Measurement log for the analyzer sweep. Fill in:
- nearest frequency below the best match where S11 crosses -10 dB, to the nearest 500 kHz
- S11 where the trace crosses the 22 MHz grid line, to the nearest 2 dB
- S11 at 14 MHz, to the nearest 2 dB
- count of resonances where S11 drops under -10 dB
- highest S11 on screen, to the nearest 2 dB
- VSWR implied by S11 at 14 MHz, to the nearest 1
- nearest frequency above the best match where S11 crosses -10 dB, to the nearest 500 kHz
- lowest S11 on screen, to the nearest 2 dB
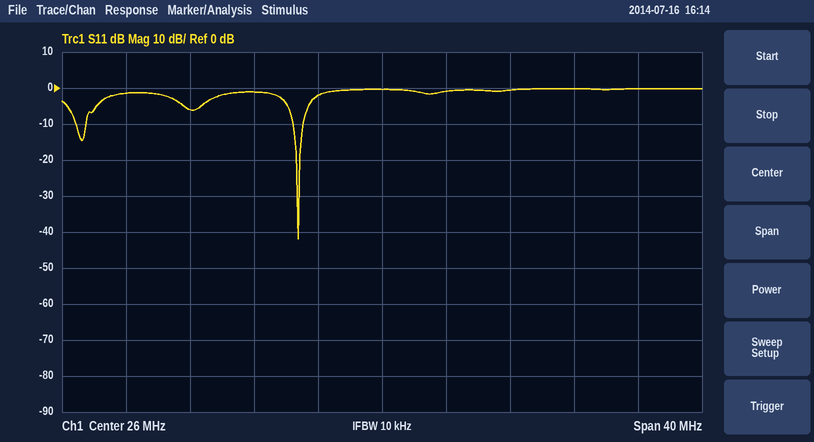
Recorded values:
20.5 MHz
-2 dB
-6 dB
2
0 dB
3
21.0 MHz
-42 dB
